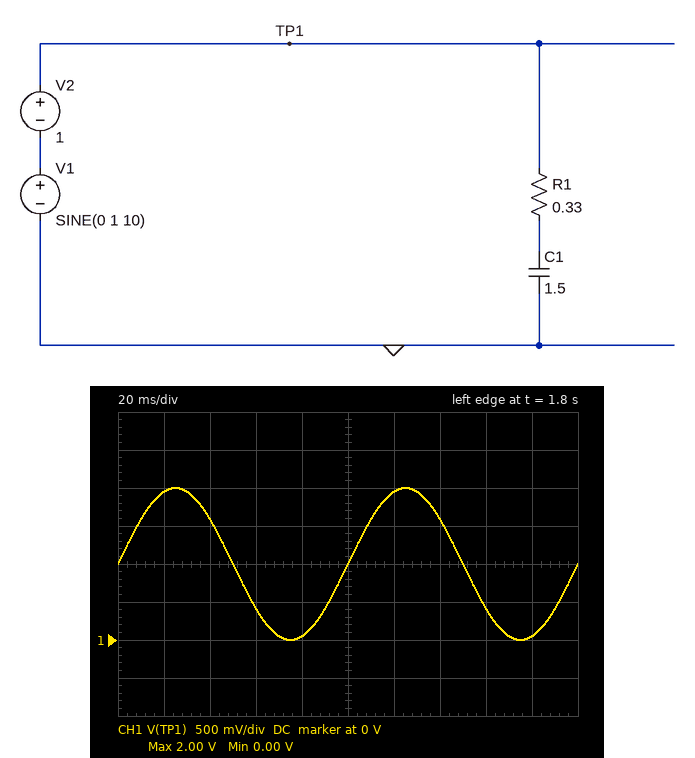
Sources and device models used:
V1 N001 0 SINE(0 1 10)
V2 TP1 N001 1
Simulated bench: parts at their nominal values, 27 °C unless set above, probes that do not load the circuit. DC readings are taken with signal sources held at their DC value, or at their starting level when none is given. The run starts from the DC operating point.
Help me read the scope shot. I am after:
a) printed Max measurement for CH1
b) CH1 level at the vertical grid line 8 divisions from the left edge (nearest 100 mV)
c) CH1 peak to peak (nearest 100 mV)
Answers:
2.00 V
400 mV
2.0 V
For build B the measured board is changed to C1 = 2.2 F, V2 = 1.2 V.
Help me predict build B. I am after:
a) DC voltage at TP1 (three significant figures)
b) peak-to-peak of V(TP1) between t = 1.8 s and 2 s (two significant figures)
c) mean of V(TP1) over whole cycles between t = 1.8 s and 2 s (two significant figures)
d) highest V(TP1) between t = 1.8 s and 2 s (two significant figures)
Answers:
1.20 V
2.0 V
1.2 V
2.2 V
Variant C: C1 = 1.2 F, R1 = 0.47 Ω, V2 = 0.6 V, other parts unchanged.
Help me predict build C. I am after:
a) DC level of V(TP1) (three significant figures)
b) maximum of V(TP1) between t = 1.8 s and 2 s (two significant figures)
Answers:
600 mV
1.6 V
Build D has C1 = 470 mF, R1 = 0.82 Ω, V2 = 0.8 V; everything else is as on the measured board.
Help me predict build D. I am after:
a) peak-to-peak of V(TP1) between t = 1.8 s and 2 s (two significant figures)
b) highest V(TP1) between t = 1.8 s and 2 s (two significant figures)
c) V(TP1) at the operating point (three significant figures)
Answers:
2.0 V
1.8 V
800 mV
